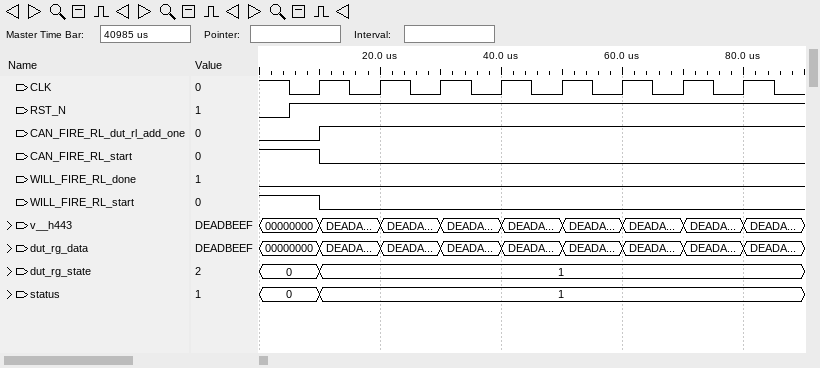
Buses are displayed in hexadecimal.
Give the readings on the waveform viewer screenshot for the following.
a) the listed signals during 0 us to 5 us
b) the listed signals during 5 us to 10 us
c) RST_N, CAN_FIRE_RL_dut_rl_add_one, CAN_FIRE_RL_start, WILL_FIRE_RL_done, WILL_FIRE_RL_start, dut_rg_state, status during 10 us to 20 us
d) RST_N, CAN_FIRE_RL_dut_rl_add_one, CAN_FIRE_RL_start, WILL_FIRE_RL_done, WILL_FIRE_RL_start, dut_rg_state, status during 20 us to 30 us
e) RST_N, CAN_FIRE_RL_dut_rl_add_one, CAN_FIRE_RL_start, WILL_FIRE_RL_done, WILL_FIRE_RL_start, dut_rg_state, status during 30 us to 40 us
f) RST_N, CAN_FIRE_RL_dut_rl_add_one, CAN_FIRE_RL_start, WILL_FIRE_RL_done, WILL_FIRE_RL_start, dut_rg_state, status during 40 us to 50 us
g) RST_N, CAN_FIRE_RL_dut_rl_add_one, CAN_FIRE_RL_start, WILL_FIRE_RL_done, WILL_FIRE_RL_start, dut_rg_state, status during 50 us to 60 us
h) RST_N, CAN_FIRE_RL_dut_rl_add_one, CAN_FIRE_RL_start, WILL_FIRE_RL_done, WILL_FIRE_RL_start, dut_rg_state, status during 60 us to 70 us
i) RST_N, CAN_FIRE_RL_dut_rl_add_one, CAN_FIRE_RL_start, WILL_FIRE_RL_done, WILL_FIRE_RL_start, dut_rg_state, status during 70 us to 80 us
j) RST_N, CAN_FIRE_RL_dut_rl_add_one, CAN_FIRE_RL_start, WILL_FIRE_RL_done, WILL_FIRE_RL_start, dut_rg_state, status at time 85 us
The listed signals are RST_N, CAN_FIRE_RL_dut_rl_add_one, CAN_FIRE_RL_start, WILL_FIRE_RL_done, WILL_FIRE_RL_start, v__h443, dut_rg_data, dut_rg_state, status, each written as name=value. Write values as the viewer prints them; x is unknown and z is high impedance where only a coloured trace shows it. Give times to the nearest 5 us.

RST_N=0, CAN_FIRE_RL_dut_rl_add_one=0, CAN_FIRE_RL_start=1, WILL_FIRE_RL_done=0, WILL_FIRE_RL_start=1, v__h443=00000000, dut_rg_data=00000000, dut_rg_state=0, status=0
RST_N=1, CAN_FIRE_RL_dut_rl_add_one=0, CAN_FIRE_RL_start=1, WILL_FIRE_RL_done=0, WILL_FIRE_RL_start=1, v__h443=00000000, dut_rg_data=00000000, dut_rg_state=0, status=0
RST_N=1, CAN_FIRE_RL_dut_rl_add_one=1, CAN_FIRE_RL_start=0, WILL_FIRE_RL_done=0, WILL_FIRE_RL_start=0, dut_rg_state=1, status=1
RST_N=1, CAN_FIRE_RL_dut_rl_add_one=1, CAN_FIRE_RL_start=0, WILL_FIRE_RL_done=0, WILL_FIRE_RL_start=0, dut_rg_state=1, status=1
RST_N=1, CAN_FIRE_RL_dut_rl_add_one=1, CAN_FIRE_RL_start=0, WILL_FIRE_RL_done=0, WILL_FIRE_RL_start=0, dut_rg_state=1, status=1
RST_N=1, CAN_FIRE_RL_dut_rl_add_one=1, CAN_FIRE_RL_start=0, WILL_FIRE_RL_done=0, WILL_FIRE_RL_start=0, dut_rg_state=1, status=1
RST_N=1, CAN_FIRE_RL_dut_rl_add_one=1, CAN_FIRE_RL_start=0, WILL_FIRE_RL_done=0, WILL_FIRE_RL_start=0, dut_rg_state=1, status=1
RST_N=1, CAN_FIRE_RL_dut_rl_add_one=1, CAN_FIRE_RL_start=0, WILL_FIRE_RL_done=0, WILL_FIRE_RL_start=0, dut_rg_state=1, status=1
RST_N=1, CAN_FIRE_RL_dut_rl_add_one=1, CAN_FIRE_RL_start=0, WILL_FIRE_RL_done=0, WILL_FIRE_RL_start=0, dut_rg_state=1, status=1
RST_N=1, CAN_FIRE_RL_dut_rl_add_one=1, CAN_FIRE_RL_start=0, WILL_FIRE_RL_done=0, WILL_FIRE_RL_start=0, dut_rg_state=1, status=1
